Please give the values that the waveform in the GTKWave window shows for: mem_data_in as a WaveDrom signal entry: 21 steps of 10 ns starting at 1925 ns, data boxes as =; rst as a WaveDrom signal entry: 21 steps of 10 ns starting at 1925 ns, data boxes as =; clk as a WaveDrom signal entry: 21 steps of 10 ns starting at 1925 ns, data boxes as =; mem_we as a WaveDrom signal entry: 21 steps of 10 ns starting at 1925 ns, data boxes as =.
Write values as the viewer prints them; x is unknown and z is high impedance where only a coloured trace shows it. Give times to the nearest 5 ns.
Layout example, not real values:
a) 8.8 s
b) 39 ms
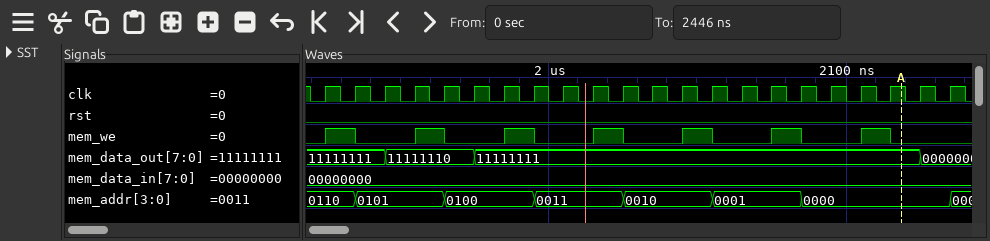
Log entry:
a) {name: 'mem_data_in', wave: '=....................', data: '00000000'}
b) {name: 'rst', wave: '0....................'}
c) {name: 'clk', wave: 'p....................'}
d) {name: 'mem_we', wave: '10.10.10.10.10.10.10.'}
